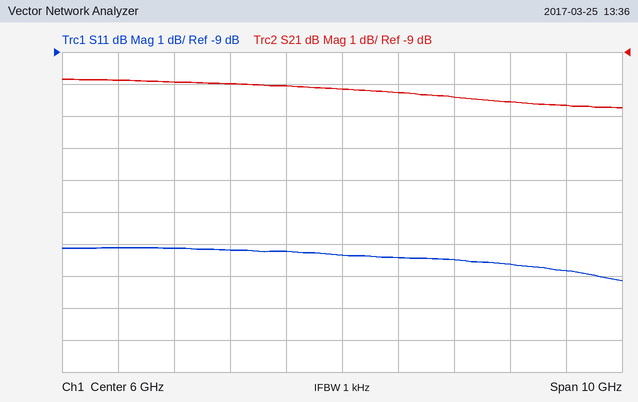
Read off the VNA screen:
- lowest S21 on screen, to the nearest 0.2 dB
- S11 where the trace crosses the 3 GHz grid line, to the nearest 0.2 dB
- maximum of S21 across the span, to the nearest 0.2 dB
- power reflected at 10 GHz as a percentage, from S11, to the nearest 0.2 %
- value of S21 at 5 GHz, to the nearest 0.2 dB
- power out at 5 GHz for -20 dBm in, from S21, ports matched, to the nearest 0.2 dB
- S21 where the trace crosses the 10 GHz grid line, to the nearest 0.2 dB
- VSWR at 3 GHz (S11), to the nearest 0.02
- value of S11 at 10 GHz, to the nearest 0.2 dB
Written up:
-10.8 dB
-15.2 dB
-9.8 dB
2.6 %
-10.0 dB
-30.0 dBm
-10.6 dB
1.42
-15.8 dB
